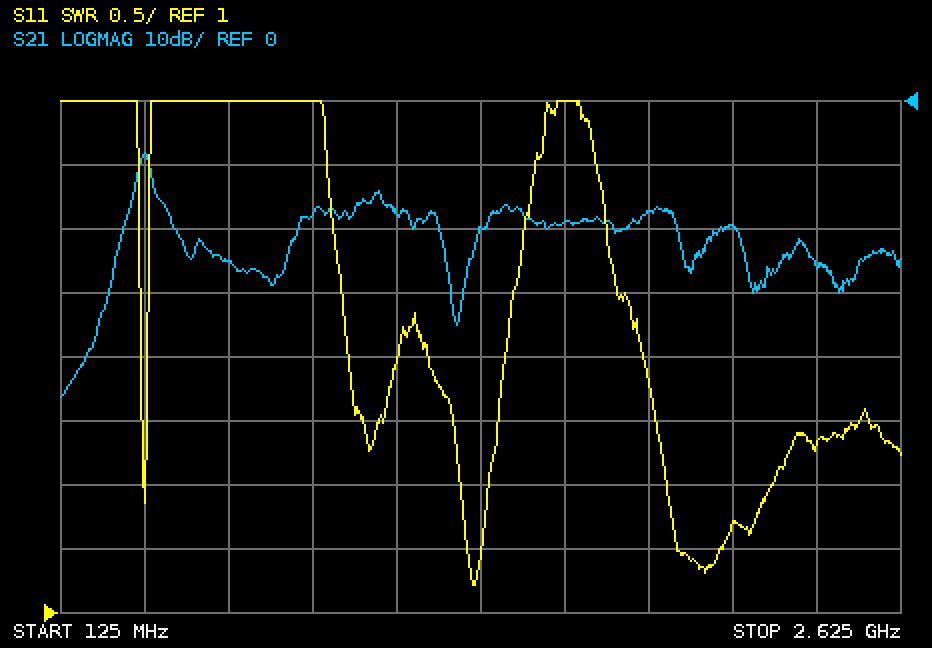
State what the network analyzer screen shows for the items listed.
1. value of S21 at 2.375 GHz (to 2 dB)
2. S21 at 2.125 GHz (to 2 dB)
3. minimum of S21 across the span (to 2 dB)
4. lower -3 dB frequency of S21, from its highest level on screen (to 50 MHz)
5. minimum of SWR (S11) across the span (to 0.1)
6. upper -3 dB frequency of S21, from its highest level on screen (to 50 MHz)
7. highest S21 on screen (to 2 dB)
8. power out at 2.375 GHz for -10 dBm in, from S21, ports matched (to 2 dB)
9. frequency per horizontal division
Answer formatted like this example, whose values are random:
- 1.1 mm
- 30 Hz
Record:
- -26 dB
- -20 dB
- -46 dB
- 350 MHz
- 1.2
- 400 MHz
- -8 dB
- -36 dBm
- 250 MHz
